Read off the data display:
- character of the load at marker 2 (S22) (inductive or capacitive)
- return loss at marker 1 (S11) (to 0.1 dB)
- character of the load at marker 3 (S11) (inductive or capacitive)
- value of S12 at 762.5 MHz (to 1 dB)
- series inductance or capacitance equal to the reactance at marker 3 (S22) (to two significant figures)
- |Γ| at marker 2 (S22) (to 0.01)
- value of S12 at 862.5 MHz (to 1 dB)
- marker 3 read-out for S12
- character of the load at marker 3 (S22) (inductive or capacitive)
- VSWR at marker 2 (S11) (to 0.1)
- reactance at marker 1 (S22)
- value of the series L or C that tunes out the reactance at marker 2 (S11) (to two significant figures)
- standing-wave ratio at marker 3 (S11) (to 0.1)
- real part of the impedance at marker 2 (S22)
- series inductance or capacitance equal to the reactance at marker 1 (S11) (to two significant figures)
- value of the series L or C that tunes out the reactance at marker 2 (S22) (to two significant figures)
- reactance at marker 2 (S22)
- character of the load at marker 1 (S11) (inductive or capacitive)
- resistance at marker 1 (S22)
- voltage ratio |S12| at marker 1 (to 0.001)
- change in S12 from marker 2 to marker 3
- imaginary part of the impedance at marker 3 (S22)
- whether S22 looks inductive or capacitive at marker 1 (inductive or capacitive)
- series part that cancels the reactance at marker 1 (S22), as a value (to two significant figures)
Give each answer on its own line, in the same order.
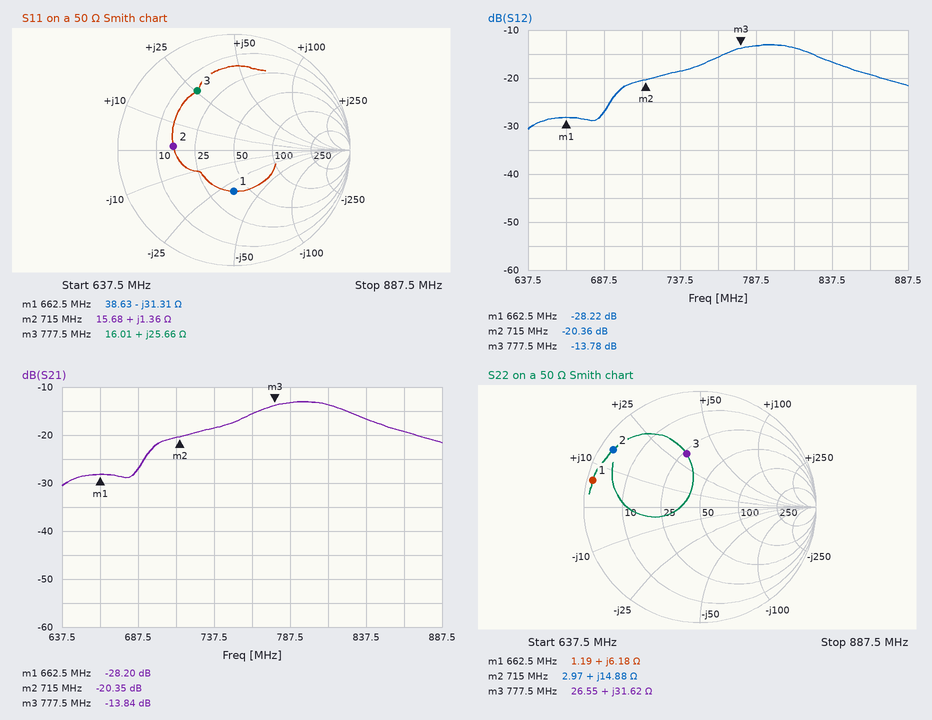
inductive
9.0 dB
inductive
-16 dB
6.5 nH
0.90
-19 dB
-13.78 dB
inductive
3.2
+6.18 Ω
160 pF
4.0
2.97 Ω
7.7 pF
15 pF
+14.88 Ω
capacitive
1.19 Ω
0.039
6.58 dB
+31.62 Ω
inductive
39 pF
